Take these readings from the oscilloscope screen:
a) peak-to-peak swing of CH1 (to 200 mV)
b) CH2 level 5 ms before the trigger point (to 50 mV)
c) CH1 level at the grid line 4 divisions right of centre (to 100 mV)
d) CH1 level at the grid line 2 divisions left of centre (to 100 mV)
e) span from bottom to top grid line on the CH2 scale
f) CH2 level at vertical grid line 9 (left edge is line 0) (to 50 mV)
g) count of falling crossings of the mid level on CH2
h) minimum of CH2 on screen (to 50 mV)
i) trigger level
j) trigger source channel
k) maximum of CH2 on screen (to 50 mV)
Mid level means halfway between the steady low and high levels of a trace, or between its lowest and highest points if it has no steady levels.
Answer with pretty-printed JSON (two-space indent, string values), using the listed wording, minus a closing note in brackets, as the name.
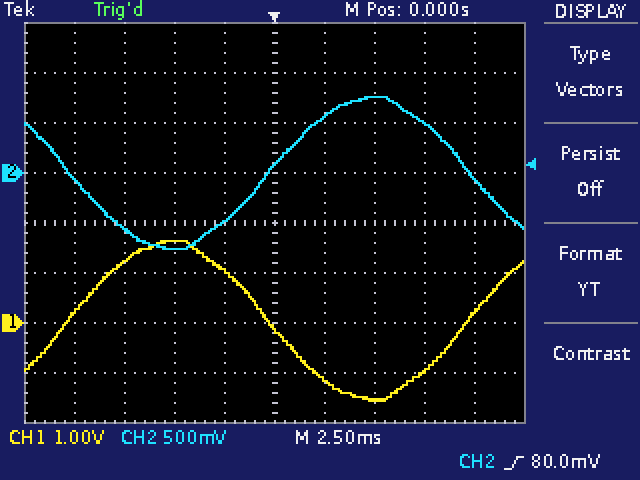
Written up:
{
  "peak-to-peak swing of CH1": "3.2 V",
  "CH2 level 5 ms before the trigger point": "-750 mV",
  "CH1 level at the grid line 4 divisions right of centre": "200 mV",
  "CH1 level at the grid line 2 divisions left of centre": "1.6 V",
  "span from bottom to top grid line on the CH2 scale": "4 V",
  "CH2 level at vertical grid line 9 (left edge is line 0)": "-50 mV",
  "count of falling crossings of the mid level on CH2": "2",
  "minimum of CH2 on screen": "-750 mV",
  "trigger level": "80.0 mV",
  "trigger source channel": "CH2",
  "maximum of CH2 on screen": "750 mV"
}
